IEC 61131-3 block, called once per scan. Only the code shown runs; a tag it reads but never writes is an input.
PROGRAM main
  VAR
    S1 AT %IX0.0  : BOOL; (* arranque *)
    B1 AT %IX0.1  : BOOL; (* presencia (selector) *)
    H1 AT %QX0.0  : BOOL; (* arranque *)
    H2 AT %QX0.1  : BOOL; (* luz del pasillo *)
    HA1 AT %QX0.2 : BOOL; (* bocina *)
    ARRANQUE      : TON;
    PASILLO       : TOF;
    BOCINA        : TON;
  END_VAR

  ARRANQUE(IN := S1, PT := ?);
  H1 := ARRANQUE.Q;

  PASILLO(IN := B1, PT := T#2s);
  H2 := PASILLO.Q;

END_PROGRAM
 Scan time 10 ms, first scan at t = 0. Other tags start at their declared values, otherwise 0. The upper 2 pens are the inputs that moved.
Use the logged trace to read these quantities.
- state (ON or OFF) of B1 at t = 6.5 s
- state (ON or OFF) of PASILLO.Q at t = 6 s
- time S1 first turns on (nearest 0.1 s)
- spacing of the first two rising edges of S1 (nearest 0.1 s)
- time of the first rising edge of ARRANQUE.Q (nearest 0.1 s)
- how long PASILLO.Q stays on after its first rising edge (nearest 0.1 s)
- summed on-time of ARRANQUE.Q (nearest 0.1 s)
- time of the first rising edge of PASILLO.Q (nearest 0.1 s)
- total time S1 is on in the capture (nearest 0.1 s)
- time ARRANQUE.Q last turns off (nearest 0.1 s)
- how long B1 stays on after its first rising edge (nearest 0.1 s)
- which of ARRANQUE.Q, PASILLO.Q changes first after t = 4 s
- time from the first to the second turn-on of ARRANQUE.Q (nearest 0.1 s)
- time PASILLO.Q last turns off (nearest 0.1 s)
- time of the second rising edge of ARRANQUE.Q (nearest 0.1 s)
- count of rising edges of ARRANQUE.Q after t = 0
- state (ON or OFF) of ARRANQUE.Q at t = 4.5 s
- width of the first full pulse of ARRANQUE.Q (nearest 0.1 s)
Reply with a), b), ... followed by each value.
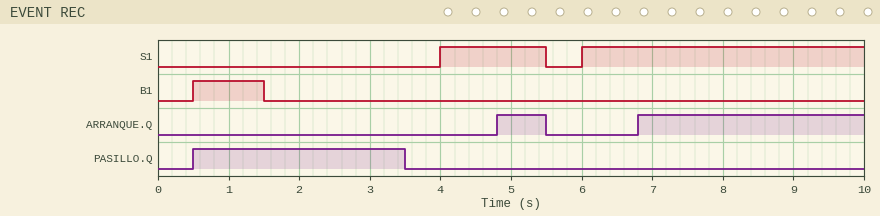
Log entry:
a) OFF
b) OFF
c) 4.0 s
d) 2.0 s
e) 4.8 s
f) 3.0 s
g) 3.9 s
h) 0.5 s
i) 5.5 s
j) 5.5 s
k) 1.0 s
l) ARRANQUE.Q
m) 2.0 s
n) 3.5 s
o) 6.8 s
p) 2
q) OFF
r) 0.7 s
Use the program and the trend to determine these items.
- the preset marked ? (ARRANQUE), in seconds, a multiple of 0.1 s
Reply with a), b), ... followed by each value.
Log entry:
a) 0.8 s
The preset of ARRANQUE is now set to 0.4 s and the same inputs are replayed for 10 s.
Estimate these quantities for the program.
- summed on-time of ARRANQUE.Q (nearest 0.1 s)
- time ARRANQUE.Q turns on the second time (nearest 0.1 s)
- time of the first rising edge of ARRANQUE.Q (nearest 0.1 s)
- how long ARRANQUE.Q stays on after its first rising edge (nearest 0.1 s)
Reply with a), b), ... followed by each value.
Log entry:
a) 4.7 s
b) 6.4 s
c) 4.4 s
d) 1.1 s
